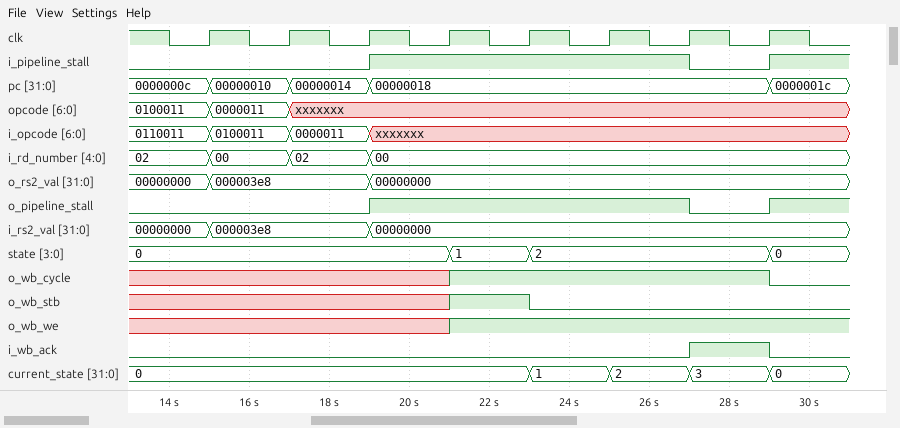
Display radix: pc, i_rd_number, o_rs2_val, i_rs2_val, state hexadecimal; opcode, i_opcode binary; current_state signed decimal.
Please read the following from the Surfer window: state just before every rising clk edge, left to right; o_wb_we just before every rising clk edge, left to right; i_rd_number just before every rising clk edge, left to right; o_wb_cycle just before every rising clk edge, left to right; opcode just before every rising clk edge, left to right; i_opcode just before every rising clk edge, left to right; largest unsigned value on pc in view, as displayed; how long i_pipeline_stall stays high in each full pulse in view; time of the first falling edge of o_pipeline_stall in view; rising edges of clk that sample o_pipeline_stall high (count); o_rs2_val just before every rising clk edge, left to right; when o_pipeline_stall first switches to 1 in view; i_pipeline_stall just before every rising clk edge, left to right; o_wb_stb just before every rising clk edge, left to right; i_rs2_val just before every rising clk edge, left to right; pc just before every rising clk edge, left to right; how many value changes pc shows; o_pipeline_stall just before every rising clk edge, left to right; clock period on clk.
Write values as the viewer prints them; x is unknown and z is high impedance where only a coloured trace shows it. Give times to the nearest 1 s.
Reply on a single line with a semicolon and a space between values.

0, 0, 0, 0, 1, 2, 2, 2; x x x x 1 1 1 1; 02, 00, 02, 00, 00, 00, 00, 00; x x x x 1 1 1 1; 0100011, 0000011, xxxxxxx, xxxxxxx, xxxxxxx, xxxxxxx, xxxxxxx, xxxxxxx; 0110011, 0100011, 0000011, xxxxxxx, xxxxxxx, xxxxxxx, xxxxxxx, xxxxxxx; 0000001c; 8 s; 27 s; 4; 00000000, 000003e8, 000003e8, 00000000, 00000000, 00000000, 00000000, 00000000; 19 s; 0 0 0 1 1 1 1 0; x x x x 1 0 0 0; 00000000, 000003e8, 000003e8, 00000000, 00000000, 00000000, 00000000, 00000000; 0000000c, 00000010, 00000014, 00000018, 00000018, 00000018, 00000018, 00000018; 4; 0 0 0 1 1 1 1 0; 2 s
